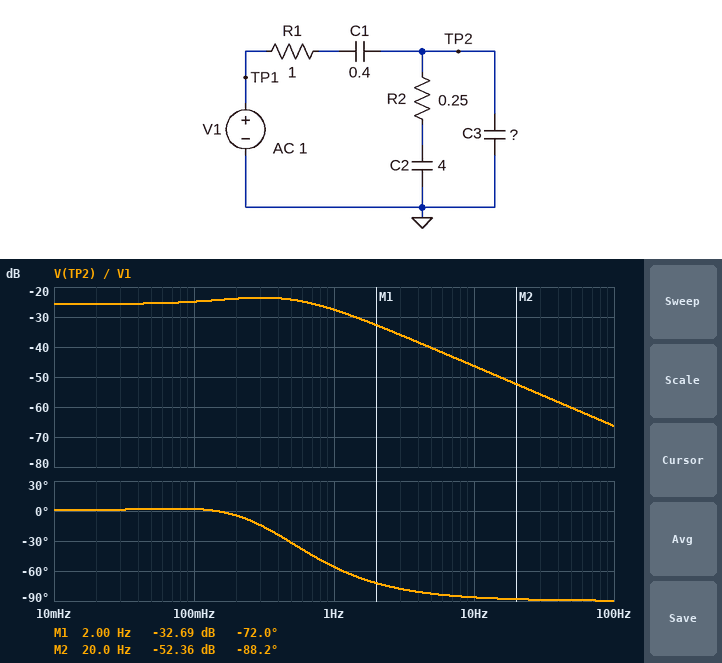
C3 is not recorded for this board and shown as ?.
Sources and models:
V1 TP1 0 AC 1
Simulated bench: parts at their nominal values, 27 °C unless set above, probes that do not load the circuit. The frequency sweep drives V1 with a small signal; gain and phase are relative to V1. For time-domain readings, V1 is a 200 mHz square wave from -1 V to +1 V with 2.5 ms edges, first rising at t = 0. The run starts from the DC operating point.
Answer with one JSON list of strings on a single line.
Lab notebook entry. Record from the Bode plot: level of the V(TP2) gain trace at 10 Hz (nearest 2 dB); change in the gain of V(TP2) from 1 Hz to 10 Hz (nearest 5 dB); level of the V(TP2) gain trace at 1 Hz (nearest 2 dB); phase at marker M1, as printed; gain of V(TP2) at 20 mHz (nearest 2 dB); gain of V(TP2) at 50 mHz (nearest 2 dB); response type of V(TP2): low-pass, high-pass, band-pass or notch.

["-46 dB", "-20 dB", "-28 dB", "-72.0 deg", "-26 dB", "-26 dB", "low-pass"]
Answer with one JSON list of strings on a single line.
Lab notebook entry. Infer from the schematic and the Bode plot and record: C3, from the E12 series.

["3.3 F"]
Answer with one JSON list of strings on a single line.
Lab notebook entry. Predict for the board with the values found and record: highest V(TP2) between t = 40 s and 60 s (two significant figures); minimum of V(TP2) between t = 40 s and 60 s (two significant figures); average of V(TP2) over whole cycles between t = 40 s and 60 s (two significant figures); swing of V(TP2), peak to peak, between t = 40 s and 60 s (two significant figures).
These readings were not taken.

["130 mV", "-23 mV", "52 mV", "150 mV"]
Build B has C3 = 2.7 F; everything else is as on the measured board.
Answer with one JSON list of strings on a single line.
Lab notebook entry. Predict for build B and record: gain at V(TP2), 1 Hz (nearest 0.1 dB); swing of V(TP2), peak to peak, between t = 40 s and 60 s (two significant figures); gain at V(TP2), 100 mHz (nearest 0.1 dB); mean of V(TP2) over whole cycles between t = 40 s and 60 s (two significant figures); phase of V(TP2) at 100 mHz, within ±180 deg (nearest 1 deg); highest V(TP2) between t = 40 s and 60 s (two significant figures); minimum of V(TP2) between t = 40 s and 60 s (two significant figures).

["-26.0 dB", "170 mV", "-24.1 dB", "56 mV", "4 deg", "140 mV", "-29 mV"]
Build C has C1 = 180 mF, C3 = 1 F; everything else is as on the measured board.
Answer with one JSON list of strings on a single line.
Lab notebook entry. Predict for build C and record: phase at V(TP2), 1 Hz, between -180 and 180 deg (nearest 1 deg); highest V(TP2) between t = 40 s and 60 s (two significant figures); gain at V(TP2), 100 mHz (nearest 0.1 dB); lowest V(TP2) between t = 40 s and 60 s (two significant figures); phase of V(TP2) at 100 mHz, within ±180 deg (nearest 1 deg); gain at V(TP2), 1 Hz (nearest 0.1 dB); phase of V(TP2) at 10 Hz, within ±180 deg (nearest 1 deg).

["-17 deg", "150 mV", "-27.9 dB", "-81 mV", "18 deg", "-21.2 dB", "-80 deg"]
